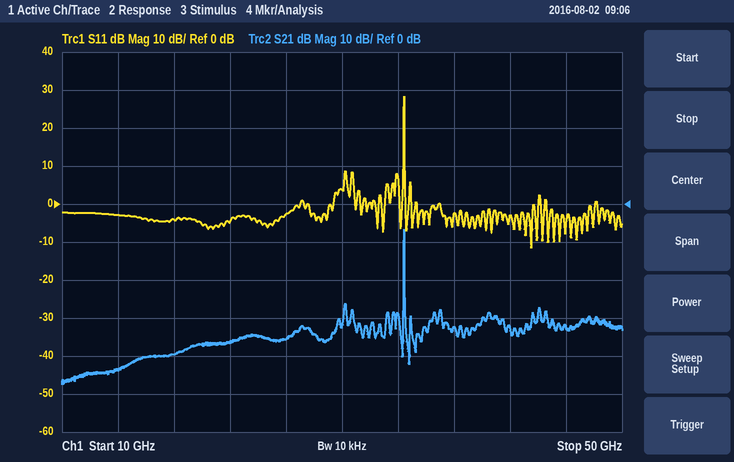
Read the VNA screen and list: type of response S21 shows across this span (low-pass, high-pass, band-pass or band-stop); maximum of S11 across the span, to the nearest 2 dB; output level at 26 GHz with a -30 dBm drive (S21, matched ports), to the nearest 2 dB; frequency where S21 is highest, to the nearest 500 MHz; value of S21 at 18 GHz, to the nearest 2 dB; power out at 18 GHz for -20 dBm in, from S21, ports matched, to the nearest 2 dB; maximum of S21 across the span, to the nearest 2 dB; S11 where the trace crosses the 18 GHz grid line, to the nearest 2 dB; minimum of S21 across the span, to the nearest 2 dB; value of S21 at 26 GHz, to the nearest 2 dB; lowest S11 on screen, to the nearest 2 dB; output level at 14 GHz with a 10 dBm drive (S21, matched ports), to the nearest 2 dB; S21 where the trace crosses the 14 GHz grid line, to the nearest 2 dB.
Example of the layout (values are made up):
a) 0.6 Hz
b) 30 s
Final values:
a) band-pass
b) 28 dB
c) -66 dBm
d) 34.5 GHz
e) -40 dB
f) -60 dBm
g) -6 dB
h) -4 dB
i) -48 dB
j) -36 dB
k) -12 dB
l) -34 dBm
m) -44 dB
